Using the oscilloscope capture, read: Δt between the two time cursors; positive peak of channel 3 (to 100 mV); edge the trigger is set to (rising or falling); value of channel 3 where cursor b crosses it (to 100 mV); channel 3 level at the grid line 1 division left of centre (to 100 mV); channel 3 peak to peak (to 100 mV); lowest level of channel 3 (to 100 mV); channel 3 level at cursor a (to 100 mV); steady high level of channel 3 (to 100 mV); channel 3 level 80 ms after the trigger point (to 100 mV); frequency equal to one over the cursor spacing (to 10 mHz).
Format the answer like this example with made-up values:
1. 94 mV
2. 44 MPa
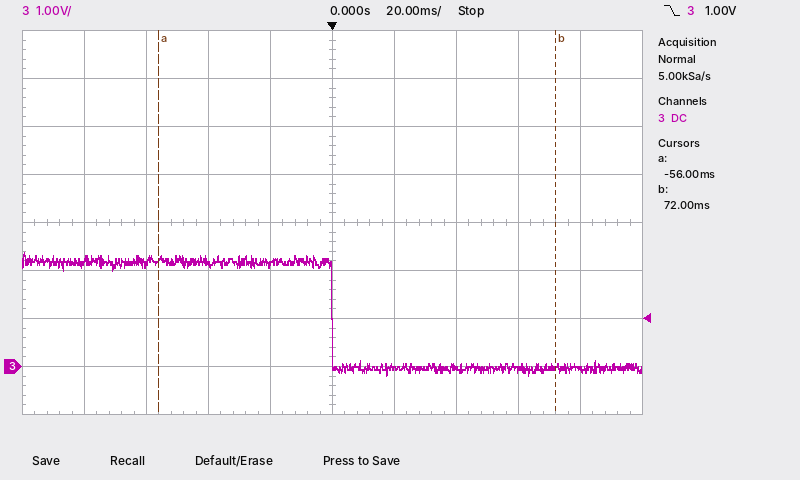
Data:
1. 128 ms
2. 2.4 V
3. falling
4. 0.0 V
5. 2.1 V
6. 2.6 V
7. -200 mV
8. 2.2 V
9. 2.2 V
10. -100 mV
11. 7.81 Hz
